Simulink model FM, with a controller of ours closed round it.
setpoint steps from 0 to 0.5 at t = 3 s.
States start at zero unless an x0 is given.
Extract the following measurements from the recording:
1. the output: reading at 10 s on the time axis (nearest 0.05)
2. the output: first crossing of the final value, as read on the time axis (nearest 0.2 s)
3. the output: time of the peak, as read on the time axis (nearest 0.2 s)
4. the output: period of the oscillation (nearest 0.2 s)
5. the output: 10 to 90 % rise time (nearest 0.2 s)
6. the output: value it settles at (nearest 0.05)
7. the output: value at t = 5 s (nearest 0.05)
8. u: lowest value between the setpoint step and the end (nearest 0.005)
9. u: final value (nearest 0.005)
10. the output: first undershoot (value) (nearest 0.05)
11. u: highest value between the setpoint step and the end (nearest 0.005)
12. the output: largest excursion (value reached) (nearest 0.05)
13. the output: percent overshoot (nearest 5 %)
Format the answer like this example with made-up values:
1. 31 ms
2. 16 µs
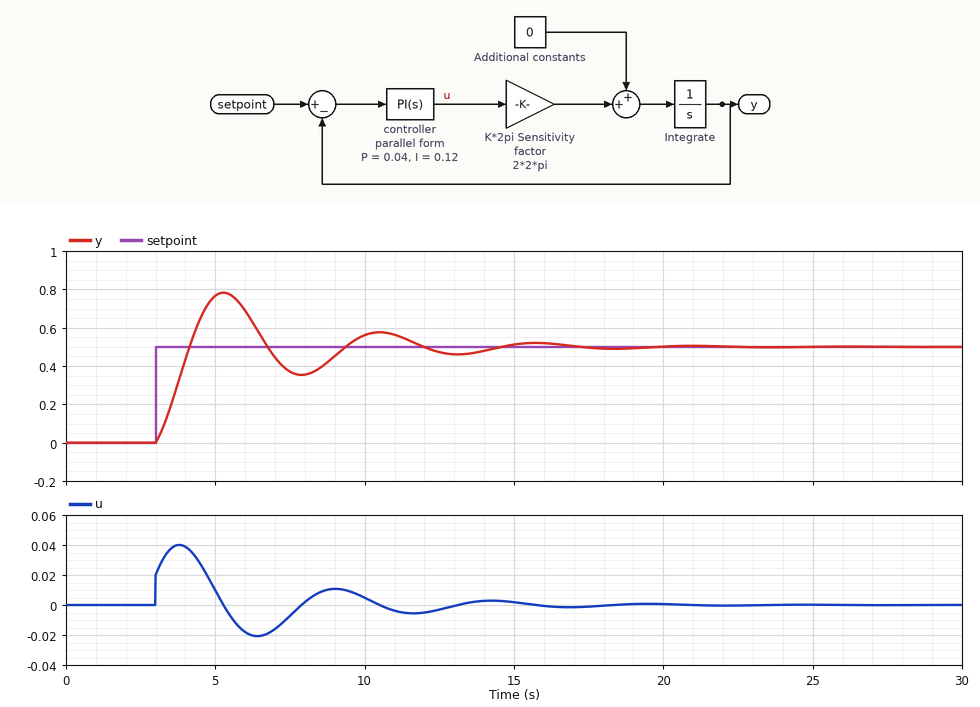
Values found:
1. 0.55
2. 4.2 s
3. 5.2 s
4. 5.2 s
5. 0.8 s
6. 0.50
7. 0.75
8. -0.020
9. 0.000
10. 0.35
11. 0.040
12. 0.80
13. 55 %
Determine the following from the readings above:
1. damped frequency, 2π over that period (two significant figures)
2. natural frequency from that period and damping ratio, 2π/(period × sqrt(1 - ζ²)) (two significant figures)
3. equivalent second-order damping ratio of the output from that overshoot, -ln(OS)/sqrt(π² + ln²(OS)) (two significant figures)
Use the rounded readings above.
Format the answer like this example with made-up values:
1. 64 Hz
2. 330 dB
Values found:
1. 1.2 rad/s
2. 1.2 rad/s
3. 0.19
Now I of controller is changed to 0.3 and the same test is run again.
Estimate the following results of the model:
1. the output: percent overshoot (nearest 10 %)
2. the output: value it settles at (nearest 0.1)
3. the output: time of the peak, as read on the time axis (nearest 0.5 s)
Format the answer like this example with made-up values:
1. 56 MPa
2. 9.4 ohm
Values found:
1. 70 %
2. 0.5
3. 4.5 s
